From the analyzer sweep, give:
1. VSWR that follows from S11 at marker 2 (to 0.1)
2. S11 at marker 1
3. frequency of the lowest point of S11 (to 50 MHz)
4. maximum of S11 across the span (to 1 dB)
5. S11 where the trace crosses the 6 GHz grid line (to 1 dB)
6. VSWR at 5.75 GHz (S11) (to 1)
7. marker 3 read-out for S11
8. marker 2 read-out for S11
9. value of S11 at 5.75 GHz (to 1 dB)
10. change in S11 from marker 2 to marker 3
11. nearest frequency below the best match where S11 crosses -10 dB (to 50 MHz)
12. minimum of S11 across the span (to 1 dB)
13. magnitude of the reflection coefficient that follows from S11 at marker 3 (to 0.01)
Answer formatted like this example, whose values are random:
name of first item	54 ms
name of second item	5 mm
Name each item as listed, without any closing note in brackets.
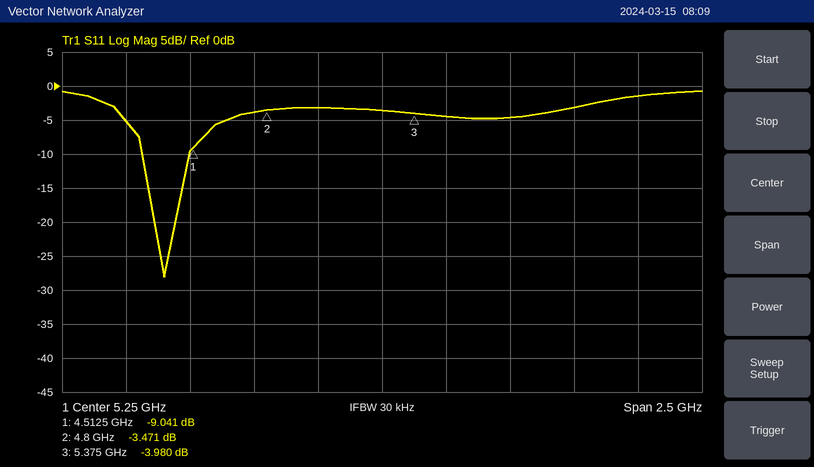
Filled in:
VSWR that follows from S11 at marker 2	5.1
S11 at marker 1	-9.041 dB
frequency of the lowest point of S11	4.40 GHz
maximum of S11 across the span	-1 dB
S11 where the trace crosses the 6 GHz grid line	-3 dB
VSWR at 5.75 GHz (S11)	4
marker 3 read-out for S11	-3.980 dB
marker 2 read-out for S11	-3.471 dB
value of S11 at 5.75 GHz	-5 dB
change in S11 from marker 2 to marker 3	-0.509 dB
nearest frequency below the best match where S11 crosses -10 dB	4.30 GHz
minimum of S11 across the span	-28 dB
magnitude of the reflection coefficient that follows from S11 at marker 3	0.63
